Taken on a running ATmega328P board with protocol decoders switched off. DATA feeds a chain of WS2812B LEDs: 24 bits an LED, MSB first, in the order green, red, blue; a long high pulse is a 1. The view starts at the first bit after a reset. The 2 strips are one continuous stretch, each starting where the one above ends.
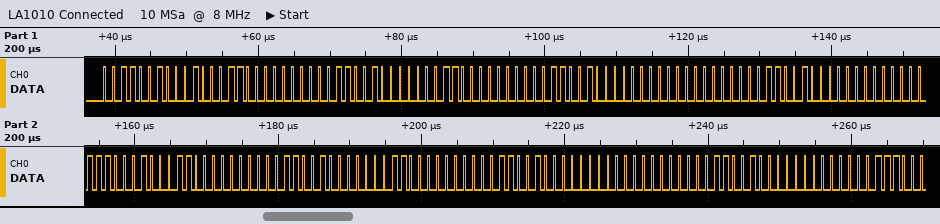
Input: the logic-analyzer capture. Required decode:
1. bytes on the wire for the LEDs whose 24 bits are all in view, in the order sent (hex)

32 23 00 32 03 00 32 00 00 32 00 0E 23 00 32 03 00 32 00 00 32
